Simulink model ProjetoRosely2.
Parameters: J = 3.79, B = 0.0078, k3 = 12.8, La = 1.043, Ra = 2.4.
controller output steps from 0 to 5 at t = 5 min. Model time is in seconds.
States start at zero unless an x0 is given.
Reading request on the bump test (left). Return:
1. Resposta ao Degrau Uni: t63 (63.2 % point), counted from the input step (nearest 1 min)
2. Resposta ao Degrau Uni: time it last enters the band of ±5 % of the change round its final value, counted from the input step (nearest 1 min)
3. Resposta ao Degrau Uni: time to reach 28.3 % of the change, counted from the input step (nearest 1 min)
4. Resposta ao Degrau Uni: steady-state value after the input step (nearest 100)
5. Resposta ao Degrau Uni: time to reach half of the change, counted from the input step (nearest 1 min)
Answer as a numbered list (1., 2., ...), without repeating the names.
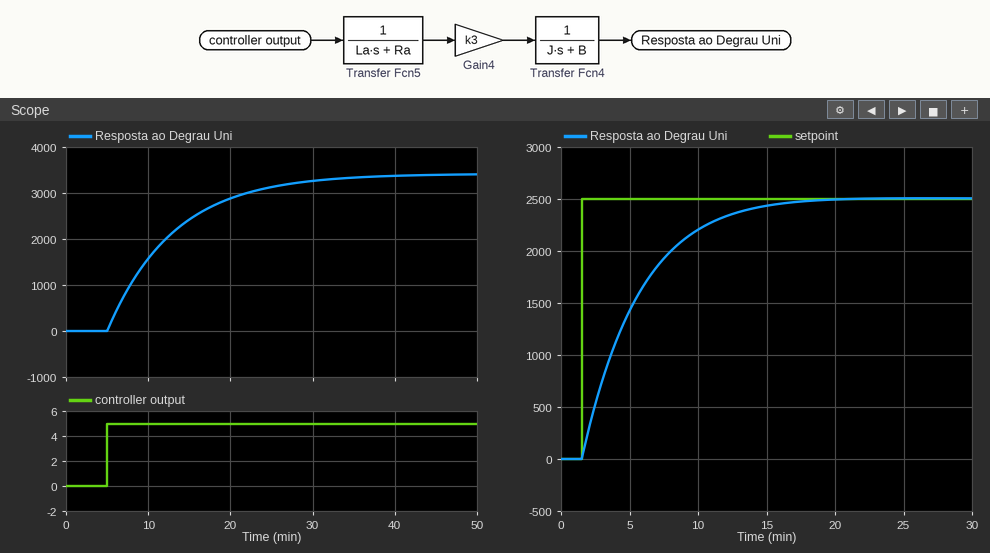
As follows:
1. 8 min
2. 24 min
3. 3 min
4. 3400
5. 6 min
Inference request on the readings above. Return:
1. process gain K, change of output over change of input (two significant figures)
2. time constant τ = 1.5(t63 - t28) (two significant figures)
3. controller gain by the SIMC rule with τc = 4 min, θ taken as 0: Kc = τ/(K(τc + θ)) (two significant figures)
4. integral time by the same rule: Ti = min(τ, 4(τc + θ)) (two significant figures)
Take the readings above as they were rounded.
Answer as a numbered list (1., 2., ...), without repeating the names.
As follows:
1. 680
2. 7.5 min
3. 0.0028
4. 7.5 min
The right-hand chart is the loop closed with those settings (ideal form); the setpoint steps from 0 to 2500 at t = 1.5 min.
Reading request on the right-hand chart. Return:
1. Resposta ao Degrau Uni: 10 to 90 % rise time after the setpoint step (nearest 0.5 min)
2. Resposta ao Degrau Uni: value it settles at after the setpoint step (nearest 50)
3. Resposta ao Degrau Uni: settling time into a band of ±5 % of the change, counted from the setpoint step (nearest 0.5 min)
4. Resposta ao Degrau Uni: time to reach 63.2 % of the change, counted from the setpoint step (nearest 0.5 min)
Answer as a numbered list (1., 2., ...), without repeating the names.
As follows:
1. 8.5 min
2. 2500
3. 11.5 min
4. 4.0 min
